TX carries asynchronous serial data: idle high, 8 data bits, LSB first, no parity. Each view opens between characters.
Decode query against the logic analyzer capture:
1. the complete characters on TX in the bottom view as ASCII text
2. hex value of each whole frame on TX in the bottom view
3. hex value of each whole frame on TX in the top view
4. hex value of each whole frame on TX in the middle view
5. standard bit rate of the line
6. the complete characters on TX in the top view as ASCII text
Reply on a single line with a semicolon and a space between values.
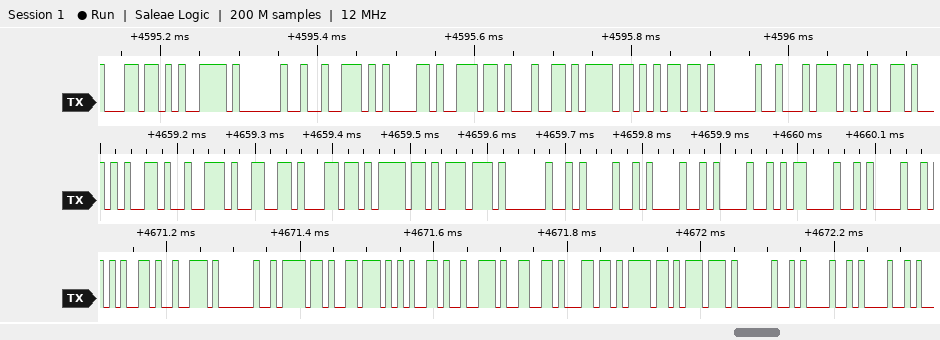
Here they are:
"er overflow !!"; 65, 72, 20, 6F, 76, 65, 72, 66, 6C, 6F, 77, 20, 21, 21; 6C, 79, 20, 72, 61, 6E, 64, 6F, 6D, 20, 74, 65; 65, 72, 66, 6C, 6F, 77, 20, 21, 21, 21, 0D, 0A; 115200 baud; "ly random te"
